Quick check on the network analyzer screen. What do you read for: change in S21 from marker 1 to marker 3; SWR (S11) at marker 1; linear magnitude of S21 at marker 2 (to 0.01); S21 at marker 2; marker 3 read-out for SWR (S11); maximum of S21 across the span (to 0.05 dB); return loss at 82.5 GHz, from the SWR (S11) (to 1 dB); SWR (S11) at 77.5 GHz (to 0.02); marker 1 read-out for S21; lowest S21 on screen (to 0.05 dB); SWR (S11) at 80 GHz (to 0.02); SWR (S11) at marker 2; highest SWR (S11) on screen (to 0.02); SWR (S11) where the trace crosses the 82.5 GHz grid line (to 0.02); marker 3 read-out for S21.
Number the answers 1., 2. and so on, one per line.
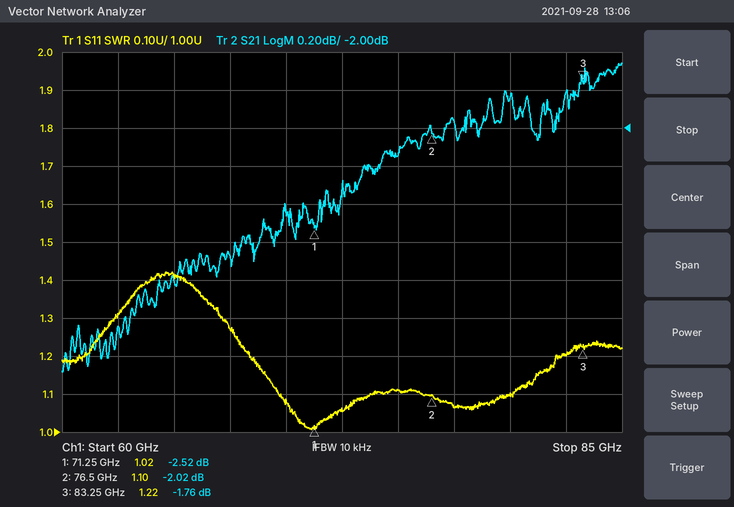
1. 0.76 dB
2. 1.02
3. 0.79
4. -2.02 dB
5. 1.22
6. -1.65 dB
7. 21 dB
8. 1.06
9. -2.52 dB
10. -3.30 dB
11. 1.10
12. 1.10
13. 1.42
14. 1.20
15. -1.76 dB
